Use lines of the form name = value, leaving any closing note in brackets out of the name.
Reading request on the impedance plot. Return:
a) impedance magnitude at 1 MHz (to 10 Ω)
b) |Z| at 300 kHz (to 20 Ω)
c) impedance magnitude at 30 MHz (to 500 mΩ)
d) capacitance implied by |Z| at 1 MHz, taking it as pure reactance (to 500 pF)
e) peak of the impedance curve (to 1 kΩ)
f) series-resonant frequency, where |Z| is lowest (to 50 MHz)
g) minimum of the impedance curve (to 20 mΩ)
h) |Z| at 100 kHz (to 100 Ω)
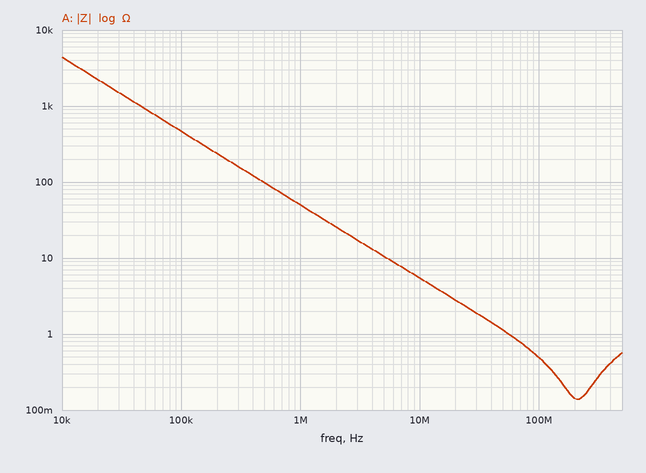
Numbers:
impedance magnitude at 1 MHz = 50 Ω
|Z| at 300 kHz = 160 Ω
impedance magnitude at 30 MHz = 2.0 Ω
capacitance implied by |Z| at 1 MHz, taking it as pure reactance = 3.0 nF
peak of the impedance curve = 4 kΩ
series-resonant frequency, where |Z| is lowest = 200 MHz
minimum of the impedance curve = 140 mΩ
|Z| at 100 kHz = 500 Ω
